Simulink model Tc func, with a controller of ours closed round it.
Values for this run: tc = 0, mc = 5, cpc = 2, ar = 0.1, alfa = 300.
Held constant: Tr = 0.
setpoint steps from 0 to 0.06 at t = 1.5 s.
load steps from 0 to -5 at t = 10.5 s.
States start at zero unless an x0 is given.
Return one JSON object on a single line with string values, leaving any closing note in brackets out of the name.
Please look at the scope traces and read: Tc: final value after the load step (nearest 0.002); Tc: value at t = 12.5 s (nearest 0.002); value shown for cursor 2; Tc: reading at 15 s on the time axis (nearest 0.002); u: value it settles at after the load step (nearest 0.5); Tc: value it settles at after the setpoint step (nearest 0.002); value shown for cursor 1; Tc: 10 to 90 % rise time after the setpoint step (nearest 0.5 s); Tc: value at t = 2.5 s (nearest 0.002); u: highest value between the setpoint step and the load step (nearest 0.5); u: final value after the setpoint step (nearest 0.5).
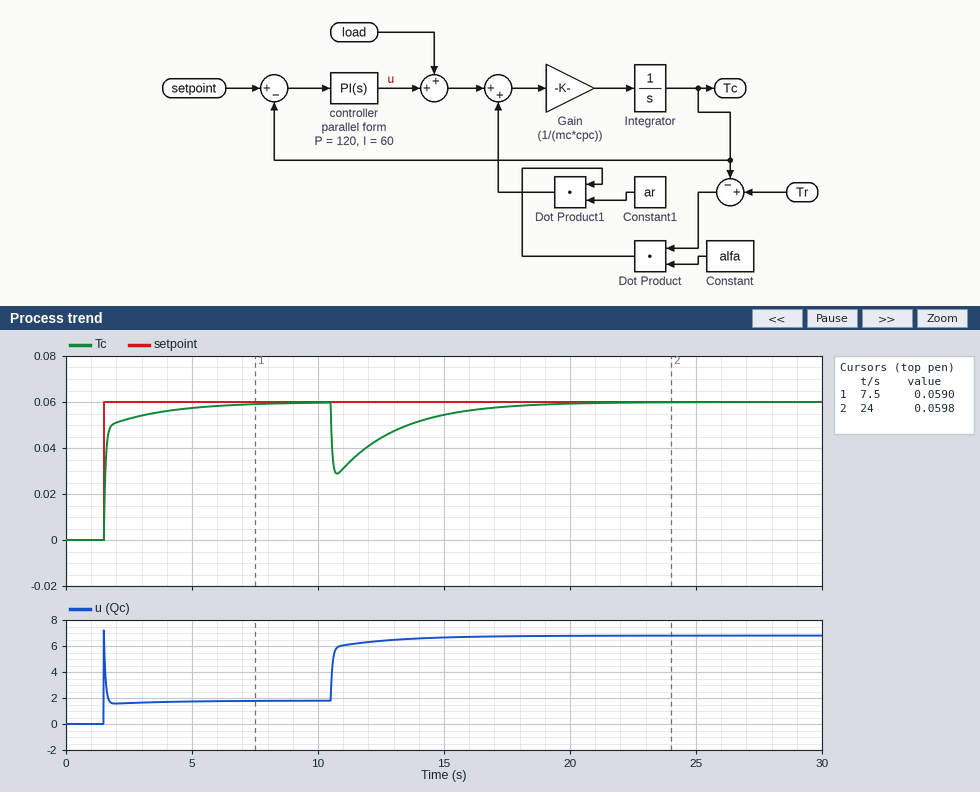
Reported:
{"Tc: final value after the load step": "0.060", "Tc: value at t = 12.5 s": "0.044", "value shown for cursor 2": "0.0598", "Tc: reading at 15 s on the time axis": "0.054", "u: value it settles at after the load step": "7.0", "Tc: value it settles at after the setpoint step": "0.060", "value shown for cursor 1": "0.0590", "Tc: 10 to 90 % rise time after the setpoint step": "1.5 s", "Tc: value at t = 2.5 s": "0.052", "u: highest value between the setpoint step and the load step": "7.0", "u: final value after the setpoint step": "2.0"}
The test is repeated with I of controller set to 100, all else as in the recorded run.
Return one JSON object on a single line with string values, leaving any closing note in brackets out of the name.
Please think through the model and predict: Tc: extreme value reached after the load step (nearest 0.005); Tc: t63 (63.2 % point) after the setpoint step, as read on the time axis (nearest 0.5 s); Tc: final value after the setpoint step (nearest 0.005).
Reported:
{"Tc: extreme value reached after the load step": "0.030", "Tc: t63 (63.2 % point) after the setpoint step, as read on the time axis": "1.5 s", "Tc: final value after the setpoint step": "0.060"}
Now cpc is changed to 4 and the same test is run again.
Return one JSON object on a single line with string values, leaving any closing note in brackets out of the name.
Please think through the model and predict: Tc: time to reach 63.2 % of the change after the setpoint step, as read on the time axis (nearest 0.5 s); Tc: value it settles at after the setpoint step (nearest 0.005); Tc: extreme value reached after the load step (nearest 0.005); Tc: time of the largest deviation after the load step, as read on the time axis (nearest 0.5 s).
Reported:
{"Tc: time to reach 63.2 % of the change after the setpoint step, as read on the time axis": "1.5 s", "Tc: value it settles at after the setpoint step": "0.060", "Tc: extreme value reached after the load step": "0.030", "Tc: time of the largest deviation after the load step, as read on the time axis": "11.0 s"}
